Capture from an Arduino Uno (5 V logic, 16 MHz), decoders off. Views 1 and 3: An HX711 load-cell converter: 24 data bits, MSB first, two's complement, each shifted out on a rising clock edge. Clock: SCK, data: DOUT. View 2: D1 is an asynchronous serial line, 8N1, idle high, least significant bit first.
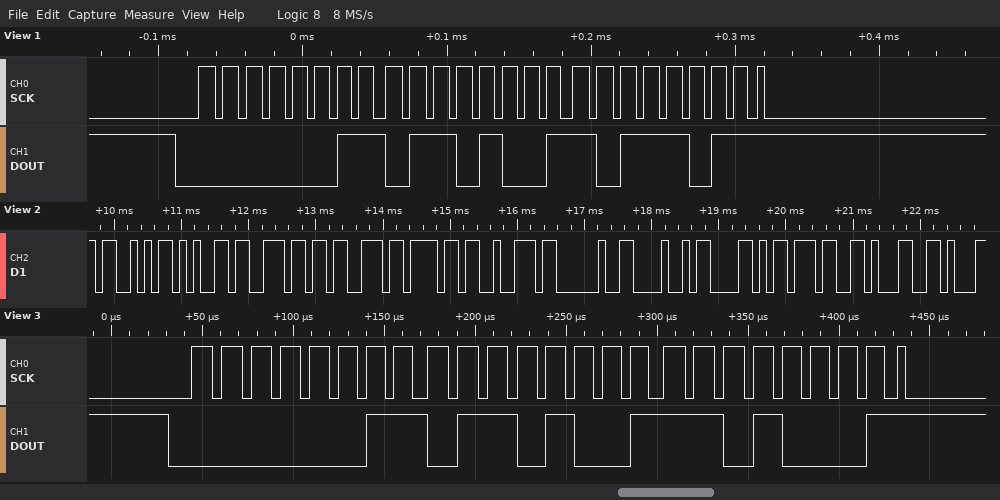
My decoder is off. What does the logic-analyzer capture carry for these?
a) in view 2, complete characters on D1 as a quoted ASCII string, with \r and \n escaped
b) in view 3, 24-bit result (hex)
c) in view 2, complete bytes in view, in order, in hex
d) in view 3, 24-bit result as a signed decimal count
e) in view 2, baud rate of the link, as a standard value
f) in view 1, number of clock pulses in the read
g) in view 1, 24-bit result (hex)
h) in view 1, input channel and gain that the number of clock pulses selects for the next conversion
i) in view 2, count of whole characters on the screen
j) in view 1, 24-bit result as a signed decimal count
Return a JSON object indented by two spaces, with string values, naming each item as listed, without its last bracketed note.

{
  "in view 2, complete characters on D1 as a quoted ASCII string, with \\r and \\n escaped": "\"Sensor HX71\"",
  "in view 3, 24-bit result": "0x0369D1",
  "in view 2, complete bytes in view, in order, in hex": "0x53 0x65 0x6E 0x73 0x6F 0x72 0x20 0x48 0x58 0x37 0x31",
  "in view 3, 24-bit result as a signed decimal count": "223697",
  "in view 2, baud rate of the link, as a standard value": "9600 baud",
  "in view 1, number of clock pulses in the read": "25",
  "in view 1, 24-bit result": "0x0369BB",
  "in view 1, input channel and gain that the number of clock pulses selects for the next conversion": "channel A, gain 128",
  "in view 2, count of whole characters on the screen": "11",
  "in view 1, 24-bit result as a signed decimal count": "223675"
}
